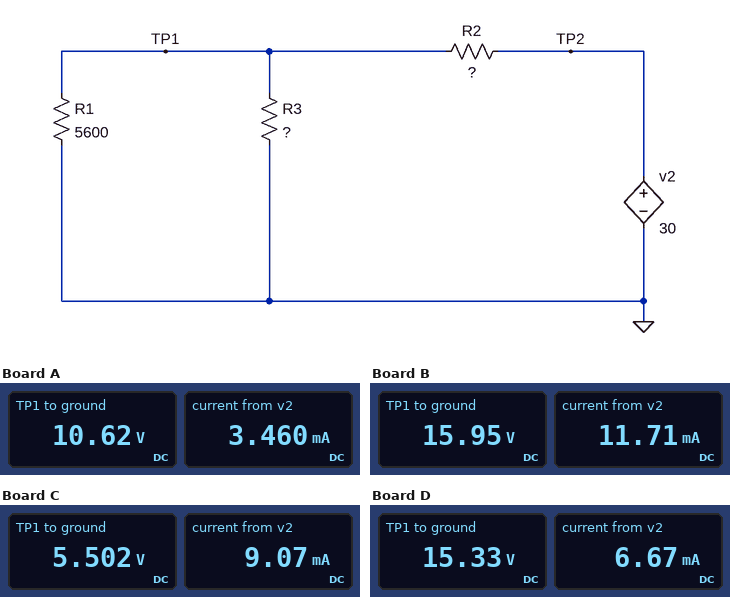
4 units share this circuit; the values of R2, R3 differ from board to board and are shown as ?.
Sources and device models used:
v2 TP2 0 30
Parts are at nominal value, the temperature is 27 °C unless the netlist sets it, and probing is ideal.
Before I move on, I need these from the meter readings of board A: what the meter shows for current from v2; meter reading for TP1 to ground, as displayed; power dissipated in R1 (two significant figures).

3.460 mA
10.62 V
20 mW
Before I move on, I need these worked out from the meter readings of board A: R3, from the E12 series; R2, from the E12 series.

6.8 kΩ
5.6 kΩ
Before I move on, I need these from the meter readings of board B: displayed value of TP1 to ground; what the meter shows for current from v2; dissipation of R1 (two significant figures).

15.95 V
11.71 mA
45 mW
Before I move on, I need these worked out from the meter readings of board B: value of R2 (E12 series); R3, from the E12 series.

1.2 kΩ
1.8 kΩ
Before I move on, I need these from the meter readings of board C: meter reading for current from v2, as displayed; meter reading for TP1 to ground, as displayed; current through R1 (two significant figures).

9.07 mA
5.502 V
980 µA
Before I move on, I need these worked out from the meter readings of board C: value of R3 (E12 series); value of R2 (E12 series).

680 Ω
2.7 kΩ
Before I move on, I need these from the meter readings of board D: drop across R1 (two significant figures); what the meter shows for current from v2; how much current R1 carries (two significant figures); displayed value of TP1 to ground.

15 V
6.67 mA
2.7 mA
15.33 V
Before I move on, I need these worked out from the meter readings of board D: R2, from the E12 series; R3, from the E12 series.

2.2 kΩ
3.9 kΩ
